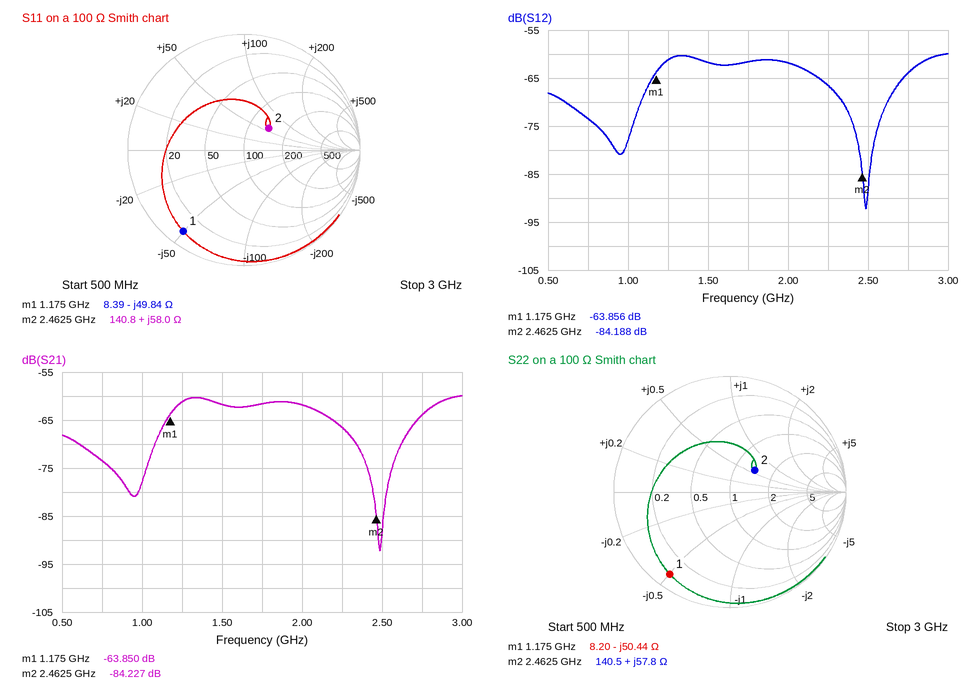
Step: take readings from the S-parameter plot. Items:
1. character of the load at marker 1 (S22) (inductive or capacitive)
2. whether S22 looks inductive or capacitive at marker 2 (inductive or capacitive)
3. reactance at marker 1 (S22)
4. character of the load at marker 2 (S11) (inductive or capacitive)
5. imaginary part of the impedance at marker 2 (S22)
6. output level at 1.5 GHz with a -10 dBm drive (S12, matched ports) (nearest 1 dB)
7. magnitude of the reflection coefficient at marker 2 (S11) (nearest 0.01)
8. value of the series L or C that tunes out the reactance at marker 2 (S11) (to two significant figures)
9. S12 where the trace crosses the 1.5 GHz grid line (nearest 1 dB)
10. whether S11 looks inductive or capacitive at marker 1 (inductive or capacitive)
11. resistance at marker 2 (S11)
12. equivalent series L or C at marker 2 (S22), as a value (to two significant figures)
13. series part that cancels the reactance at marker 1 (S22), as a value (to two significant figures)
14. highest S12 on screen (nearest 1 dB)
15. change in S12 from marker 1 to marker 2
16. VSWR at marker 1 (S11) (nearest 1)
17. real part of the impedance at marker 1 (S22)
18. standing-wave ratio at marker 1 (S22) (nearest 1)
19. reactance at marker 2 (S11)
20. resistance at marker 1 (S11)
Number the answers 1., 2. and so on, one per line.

1. capacitive
2. inductive
3. -50.44 Ω
4. inductive
5. +57.8 Ω
6. -72 dBm
7. 0.29
8. 1.1 pF
9. -62 dB
10. capacitive
11. 140.8 Ω
12. 3.7 nH
13. 6.8 nH
14. -60 dB
15. -20.332 dB
16. 15
17. 8.20 Ω
18. 15
19. +58.0 Ω
20. 8.39 Ω
